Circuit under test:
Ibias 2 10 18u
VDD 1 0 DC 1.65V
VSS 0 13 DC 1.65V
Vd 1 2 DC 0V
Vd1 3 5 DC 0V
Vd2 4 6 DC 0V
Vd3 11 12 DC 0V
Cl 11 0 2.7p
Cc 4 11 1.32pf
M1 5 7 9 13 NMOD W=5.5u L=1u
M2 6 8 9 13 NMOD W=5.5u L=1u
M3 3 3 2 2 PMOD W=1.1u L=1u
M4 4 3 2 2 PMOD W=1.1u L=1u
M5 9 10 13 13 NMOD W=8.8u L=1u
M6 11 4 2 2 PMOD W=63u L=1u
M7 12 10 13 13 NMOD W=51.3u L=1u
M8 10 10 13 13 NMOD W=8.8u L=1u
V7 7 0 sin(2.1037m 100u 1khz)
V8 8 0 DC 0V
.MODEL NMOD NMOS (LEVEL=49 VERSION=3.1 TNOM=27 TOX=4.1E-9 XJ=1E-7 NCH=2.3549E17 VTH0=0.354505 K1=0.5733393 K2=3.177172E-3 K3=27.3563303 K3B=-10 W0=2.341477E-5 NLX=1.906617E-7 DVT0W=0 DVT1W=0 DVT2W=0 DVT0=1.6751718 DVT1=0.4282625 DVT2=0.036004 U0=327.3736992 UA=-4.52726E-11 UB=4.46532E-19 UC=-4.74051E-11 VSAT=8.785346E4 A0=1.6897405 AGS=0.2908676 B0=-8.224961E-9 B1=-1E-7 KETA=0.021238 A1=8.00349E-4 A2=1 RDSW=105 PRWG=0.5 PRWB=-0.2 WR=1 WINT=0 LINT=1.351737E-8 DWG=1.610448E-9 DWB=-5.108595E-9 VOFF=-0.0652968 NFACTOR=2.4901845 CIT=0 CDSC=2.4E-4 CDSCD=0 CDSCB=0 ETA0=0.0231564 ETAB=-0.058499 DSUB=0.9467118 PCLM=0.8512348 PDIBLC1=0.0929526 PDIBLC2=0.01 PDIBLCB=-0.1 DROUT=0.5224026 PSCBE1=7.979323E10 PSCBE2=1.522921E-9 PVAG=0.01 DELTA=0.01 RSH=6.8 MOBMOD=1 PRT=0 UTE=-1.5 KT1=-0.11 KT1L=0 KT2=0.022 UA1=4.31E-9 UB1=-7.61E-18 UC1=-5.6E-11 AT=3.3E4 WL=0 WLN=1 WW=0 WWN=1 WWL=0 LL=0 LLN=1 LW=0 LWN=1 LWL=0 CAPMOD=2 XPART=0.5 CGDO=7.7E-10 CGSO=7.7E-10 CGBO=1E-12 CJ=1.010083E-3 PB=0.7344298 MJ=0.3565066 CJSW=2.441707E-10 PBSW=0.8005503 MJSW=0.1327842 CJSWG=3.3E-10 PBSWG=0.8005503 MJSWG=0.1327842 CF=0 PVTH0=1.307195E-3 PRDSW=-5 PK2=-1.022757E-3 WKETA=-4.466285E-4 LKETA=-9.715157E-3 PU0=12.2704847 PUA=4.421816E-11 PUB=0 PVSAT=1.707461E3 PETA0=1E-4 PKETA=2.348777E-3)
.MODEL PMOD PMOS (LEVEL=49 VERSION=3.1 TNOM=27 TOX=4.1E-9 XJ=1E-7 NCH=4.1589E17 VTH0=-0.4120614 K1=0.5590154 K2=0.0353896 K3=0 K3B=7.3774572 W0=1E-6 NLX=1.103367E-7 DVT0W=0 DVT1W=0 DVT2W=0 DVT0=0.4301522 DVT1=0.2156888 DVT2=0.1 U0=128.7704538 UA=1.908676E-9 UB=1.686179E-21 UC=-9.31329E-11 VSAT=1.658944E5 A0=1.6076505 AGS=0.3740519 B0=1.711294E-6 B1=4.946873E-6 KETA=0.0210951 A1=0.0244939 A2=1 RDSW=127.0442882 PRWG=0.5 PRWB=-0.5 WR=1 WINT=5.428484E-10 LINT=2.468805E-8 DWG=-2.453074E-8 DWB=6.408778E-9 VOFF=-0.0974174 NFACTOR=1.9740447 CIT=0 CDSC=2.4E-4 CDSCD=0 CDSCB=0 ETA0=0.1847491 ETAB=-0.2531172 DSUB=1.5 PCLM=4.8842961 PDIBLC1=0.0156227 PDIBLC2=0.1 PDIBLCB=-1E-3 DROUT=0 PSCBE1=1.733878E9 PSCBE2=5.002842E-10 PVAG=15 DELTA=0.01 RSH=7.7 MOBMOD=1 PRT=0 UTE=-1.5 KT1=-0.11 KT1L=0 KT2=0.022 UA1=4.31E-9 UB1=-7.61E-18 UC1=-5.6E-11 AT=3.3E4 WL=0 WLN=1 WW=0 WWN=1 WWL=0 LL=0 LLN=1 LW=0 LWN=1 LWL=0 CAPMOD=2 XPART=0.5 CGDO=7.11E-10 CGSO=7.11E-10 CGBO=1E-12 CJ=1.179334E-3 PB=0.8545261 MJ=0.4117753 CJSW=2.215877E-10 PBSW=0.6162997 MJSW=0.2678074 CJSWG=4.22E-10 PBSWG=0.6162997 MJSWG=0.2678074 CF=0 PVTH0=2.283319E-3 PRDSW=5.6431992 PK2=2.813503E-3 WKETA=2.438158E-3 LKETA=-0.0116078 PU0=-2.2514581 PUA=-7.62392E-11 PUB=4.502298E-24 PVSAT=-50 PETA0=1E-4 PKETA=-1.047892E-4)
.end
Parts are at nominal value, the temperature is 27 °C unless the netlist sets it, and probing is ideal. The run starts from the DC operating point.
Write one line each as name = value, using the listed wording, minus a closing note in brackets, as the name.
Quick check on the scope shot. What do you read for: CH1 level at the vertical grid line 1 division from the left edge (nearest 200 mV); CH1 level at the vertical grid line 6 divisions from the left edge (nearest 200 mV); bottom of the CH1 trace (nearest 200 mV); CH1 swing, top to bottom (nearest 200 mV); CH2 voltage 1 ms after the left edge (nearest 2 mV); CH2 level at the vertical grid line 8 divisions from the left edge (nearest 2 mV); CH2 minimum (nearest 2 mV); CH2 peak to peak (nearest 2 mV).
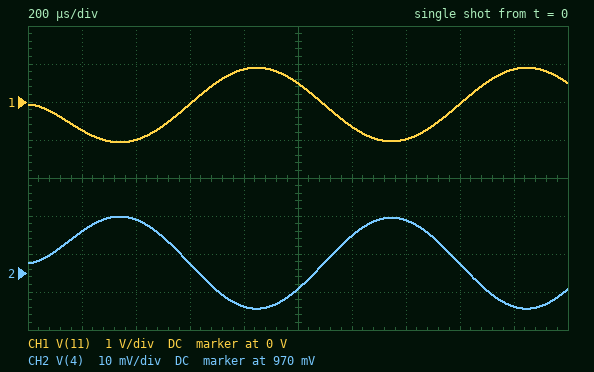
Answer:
CH1 level at the vertical grid line 1 division from the left edge = -800 mV
CH1 level at the vertical grid line 6 divisions from the left edge = -600 mV
bottom of the CH1 trace = -1.0 V
CH1 swing, top to bottom = 2.0 V
CH2 voltage 1 ms after the left edge = 966 mV
CH2 level at the vertical grid line 8 divisions from the left edge = 972 mV
CH2 minimum = 960 mV
CH2 peak to peak = 24 mV
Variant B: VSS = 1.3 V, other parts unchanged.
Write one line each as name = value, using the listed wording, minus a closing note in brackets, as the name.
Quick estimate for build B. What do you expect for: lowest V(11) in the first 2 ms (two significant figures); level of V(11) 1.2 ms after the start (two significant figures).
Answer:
lowest V(11) in the first 2 ms = -1.2 V
level of V(11) 1.2 ms after the start = -990 mV
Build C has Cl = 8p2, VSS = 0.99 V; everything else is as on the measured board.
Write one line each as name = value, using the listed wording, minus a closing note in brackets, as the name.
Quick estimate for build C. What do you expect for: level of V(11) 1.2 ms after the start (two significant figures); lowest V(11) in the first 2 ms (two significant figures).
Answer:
level of V(11) 1.2 ms after the start = -880 mV
lowest V(11) in the first 2 ms = -890 mV
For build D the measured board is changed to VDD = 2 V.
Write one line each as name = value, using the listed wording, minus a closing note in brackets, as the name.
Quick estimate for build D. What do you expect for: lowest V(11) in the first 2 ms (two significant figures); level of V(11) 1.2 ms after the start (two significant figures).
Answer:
lowest V(11) in the first 2 ms = -1.4 V
level of V(11) 1.2 ms after the start = -1.0 V
